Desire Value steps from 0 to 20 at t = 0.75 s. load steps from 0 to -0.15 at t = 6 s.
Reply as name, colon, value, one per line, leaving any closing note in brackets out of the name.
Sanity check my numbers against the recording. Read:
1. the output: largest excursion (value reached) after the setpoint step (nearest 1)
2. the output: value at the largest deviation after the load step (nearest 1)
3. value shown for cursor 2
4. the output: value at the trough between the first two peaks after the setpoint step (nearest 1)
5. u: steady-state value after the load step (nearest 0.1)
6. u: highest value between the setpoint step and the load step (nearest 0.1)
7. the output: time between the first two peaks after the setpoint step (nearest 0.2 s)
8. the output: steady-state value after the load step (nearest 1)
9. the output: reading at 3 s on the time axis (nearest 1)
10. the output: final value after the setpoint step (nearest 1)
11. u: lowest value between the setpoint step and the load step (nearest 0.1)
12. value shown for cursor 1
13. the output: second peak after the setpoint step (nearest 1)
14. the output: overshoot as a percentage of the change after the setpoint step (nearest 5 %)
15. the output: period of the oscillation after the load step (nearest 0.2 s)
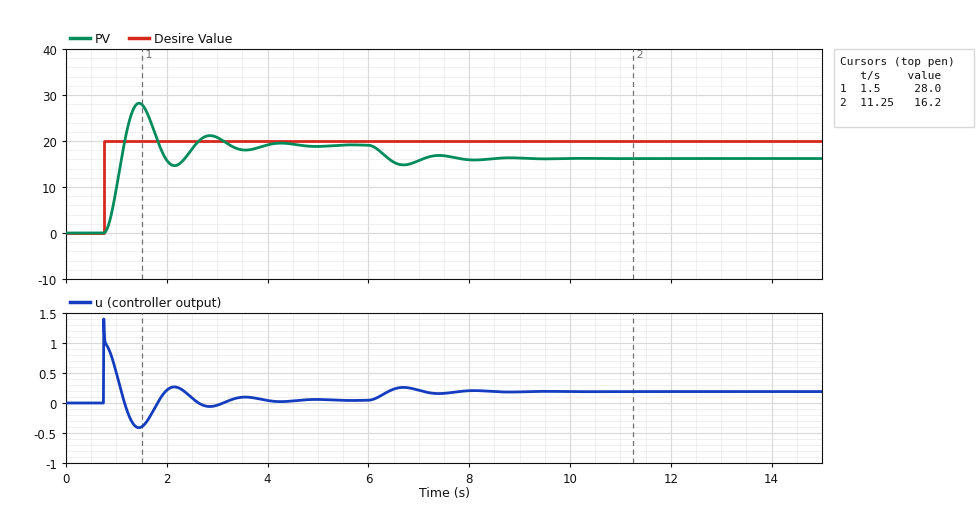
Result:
the output: largest excursion (value reached) after the setpoint step: 28
the output: value at the largest deviation after the load step: 15
value shown for cursor 2: 16.2
the output: value at the trough between the first two peaks after the setpoint step: 15
u: steady-state value after the load step: 0.2
u: highest value between the setpoint step and the load step: 1.4
the output: time between the first two peaks after the setpoint step: 1.4 s
the output: steady-state value after the load step: 16
the output: reading at 3 s on the time axis: 21
the output: final value after the setpoint step: 19
u: lowest value between the setpoint step and the load step: -0.4
value shown for cursor 1: 28.0
the output: second peak after the setpoint step: 21
the output: overshoot as a percentage of the change after the setpoint step: 50 %
the output: period of the oscillation after the load step: 1.4 s
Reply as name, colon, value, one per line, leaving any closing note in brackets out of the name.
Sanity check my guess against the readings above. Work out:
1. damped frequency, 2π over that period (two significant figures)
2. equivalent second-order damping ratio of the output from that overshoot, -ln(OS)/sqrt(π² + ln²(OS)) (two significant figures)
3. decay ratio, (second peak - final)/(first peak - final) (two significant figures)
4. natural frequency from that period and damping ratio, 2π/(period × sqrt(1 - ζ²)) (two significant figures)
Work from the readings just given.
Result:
damped frequency, 2π over that period: 4.5 rad/s
equivalent second-order damping ratio of the output from that overshoot, -ln(OS)/sqrt(π² + ln²(OS)): 0.22
decay ratio, (second peak - final)/(first peak - final): 0.22
natural frequency from that period and damping ratio, 2π/(period × sqrt(1 - ζ²)): 4.6 rad/s
